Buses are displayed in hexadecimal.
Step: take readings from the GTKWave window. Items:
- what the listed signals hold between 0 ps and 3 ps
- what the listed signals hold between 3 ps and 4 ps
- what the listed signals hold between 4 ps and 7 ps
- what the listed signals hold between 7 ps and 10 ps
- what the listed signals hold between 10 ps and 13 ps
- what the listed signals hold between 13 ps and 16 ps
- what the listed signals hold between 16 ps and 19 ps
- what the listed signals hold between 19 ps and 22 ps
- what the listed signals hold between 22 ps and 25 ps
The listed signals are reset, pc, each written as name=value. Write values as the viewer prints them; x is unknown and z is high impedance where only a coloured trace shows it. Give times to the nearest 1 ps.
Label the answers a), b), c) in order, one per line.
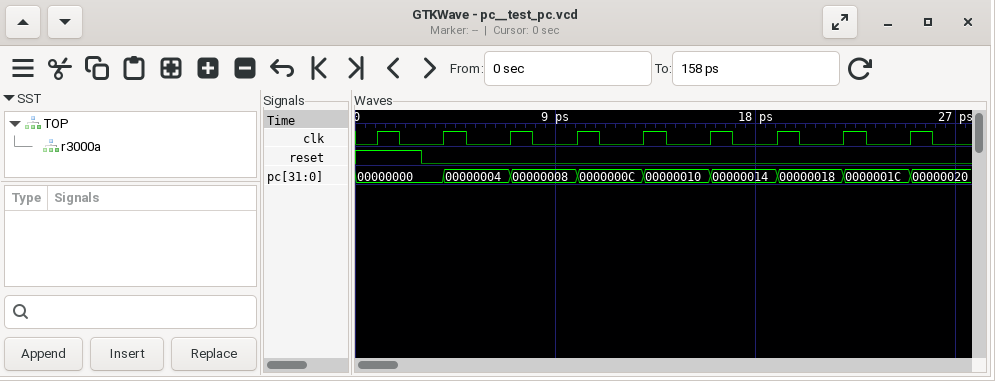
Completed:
a) reset=1, pc=00000000
b) reset=0, pc=00000000
c) reset=0, pc=00000004
d) reset=0, pc=00000008
e) reset=0, pc=0000000C
f) reset=0, pc=00000010
g) reset=0, pc=00000014
h) reset=0, pc=00000018
i) reset=0, pc=0000001C
